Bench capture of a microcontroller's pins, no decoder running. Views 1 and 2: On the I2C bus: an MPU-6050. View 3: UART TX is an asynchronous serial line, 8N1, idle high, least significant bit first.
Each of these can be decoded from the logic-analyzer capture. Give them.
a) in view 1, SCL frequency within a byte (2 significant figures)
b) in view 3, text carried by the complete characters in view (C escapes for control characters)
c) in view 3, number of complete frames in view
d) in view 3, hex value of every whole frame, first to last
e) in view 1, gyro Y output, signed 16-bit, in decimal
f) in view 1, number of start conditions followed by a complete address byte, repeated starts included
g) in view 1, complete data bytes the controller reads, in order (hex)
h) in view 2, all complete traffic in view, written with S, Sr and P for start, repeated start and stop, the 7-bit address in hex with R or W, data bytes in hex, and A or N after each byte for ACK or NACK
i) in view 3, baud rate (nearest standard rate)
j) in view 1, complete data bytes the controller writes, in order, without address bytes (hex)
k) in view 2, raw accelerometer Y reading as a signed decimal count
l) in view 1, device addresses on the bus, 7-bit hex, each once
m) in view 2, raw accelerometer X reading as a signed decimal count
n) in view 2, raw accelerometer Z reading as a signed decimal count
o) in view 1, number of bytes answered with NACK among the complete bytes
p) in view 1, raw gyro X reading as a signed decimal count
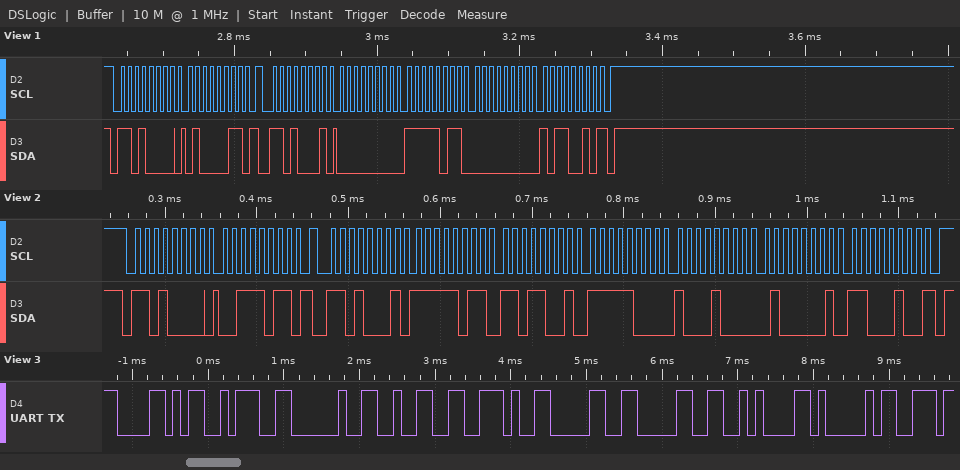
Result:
100 kHz
"X: 2.00\nA"
9
58 3A 20 32 2E 30 30 0A 41
178
2
00 FB 00 B2
S 68W A 3B A Sr 68R A FB A D9 A F8 A 88 A 41 A C4 N P
9600 baud
43
-1912
0x68
-1063
16836
1
251
